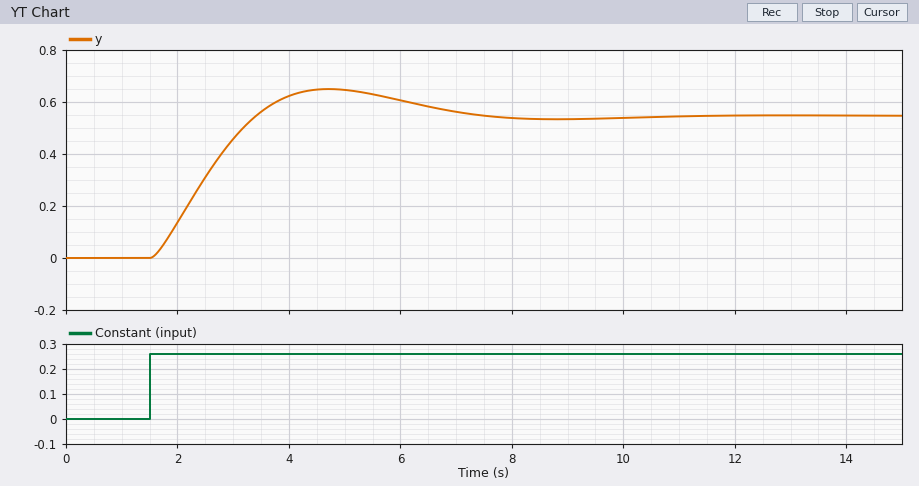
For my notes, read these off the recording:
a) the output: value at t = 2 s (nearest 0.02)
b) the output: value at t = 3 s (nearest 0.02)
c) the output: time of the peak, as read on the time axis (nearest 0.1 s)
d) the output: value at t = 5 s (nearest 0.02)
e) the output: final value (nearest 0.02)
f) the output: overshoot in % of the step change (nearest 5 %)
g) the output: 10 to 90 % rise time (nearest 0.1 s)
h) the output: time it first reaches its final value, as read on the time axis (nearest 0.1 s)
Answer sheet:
0.14
0.46
4.7 s
0.64
0.54
20 %
1.4 s
3.4 s
